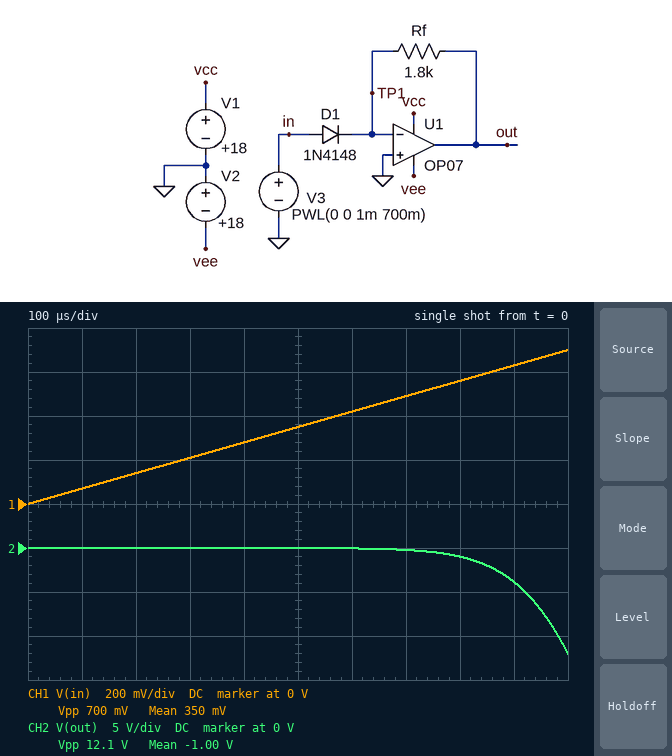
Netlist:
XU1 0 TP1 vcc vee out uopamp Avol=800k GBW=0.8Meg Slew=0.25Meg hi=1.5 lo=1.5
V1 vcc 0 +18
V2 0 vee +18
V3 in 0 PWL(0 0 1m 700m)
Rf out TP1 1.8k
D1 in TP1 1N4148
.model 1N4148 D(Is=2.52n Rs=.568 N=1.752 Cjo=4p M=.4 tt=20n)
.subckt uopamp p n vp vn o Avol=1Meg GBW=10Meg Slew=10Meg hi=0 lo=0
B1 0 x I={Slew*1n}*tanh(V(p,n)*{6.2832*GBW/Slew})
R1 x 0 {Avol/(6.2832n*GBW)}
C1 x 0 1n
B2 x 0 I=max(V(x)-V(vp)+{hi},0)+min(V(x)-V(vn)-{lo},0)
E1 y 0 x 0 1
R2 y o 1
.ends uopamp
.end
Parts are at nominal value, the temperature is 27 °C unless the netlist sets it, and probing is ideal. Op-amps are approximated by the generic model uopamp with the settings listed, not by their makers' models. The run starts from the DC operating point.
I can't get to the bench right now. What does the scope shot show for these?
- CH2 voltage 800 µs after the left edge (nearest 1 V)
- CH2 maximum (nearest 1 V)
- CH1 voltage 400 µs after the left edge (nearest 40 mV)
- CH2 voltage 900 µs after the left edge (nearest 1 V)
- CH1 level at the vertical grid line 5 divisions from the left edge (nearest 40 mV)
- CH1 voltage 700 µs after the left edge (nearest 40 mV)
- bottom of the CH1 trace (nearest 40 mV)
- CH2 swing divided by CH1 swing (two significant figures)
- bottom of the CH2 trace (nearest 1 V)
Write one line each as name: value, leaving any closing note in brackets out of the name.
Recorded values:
CH2 voltage 800 µs after the left edge: -1 V
CH2 maximum: 0 V
CH1 voltage 400 µs after the left edge: 280 mV
CH2 voltage 900 µs after the left edge: -4 V
CH1 level at the vertical grid line 5 divisions from the left edge: 360 mV
CH1 voltage 700 µs after the left edge: 480 mV
bottom of the CH1 trace: 0 V
CH2 swing divided by CH1 swing: 17
bottom of the CH2 trace: -12 V
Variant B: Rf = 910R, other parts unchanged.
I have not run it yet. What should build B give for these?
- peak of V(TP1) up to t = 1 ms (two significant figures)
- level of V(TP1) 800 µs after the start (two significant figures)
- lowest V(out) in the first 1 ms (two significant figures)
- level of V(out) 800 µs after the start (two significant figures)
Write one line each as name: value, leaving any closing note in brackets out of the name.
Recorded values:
peak of V(TP1) up to t = 1 ms: 17 mV
level of V(TP1) 800 µs after the start: 1.5 mV
lowest V(out) in the first 1 ms: -7.3 V
level of V(out) 800 µs after the start: -510 mV
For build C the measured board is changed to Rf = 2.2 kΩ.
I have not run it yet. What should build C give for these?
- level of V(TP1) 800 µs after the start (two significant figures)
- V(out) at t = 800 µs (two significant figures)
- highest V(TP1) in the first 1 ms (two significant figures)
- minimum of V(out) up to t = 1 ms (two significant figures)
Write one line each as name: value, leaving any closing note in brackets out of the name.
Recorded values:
level of V(TP1) 800 µs after the start: 3.4 mV
V(out) at t = 800 µs: -1.2 V
highest V(TP1) in the first 1 ms: 29 mV
minimum of V(out) up to t = 1 ms: -14 V
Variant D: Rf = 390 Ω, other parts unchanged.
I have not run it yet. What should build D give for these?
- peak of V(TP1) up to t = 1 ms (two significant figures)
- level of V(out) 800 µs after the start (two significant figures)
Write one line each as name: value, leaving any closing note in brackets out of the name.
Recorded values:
peak of V(TP1) up to t = 1 ms: 8.9 mV
level of V(out) 800 µs after the start: -220 mV
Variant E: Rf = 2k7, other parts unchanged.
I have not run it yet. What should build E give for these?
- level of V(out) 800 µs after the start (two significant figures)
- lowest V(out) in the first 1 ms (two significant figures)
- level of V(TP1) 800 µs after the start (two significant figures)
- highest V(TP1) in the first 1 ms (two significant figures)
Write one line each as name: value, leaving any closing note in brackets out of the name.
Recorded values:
level of V(out) 800 µs after the start: -1.4 V
lowest V(out) in the first 1 ms: -16 V
level of V(TP1) 800 µs after the start: 4.1 mV
highest V(TP1) in the first 1 ms: 33 mV
